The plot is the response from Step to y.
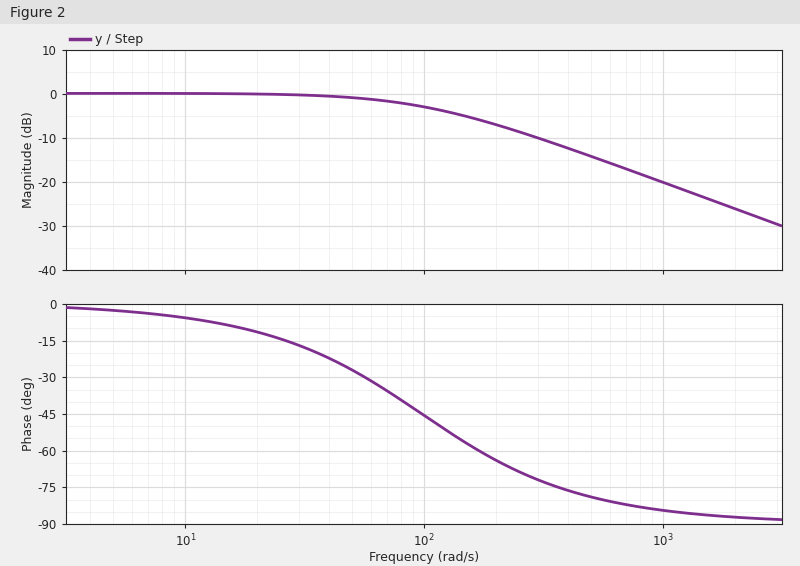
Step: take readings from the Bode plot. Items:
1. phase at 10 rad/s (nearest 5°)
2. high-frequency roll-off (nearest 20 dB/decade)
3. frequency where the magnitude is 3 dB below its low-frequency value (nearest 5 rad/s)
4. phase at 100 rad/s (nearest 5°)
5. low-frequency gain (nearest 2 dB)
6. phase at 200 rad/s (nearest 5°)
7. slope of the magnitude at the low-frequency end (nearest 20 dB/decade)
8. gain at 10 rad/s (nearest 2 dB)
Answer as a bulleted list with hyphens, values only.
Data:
- -5°
- -20 dB/decade
- 100 rad/s
- -45°
- 0 dB
- -65°
- 0 dB/decade
- 0 dB
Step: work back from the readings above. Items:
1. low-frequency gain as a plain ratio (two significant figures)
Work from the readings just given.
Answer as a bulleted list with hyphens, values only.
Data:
- 1.0
